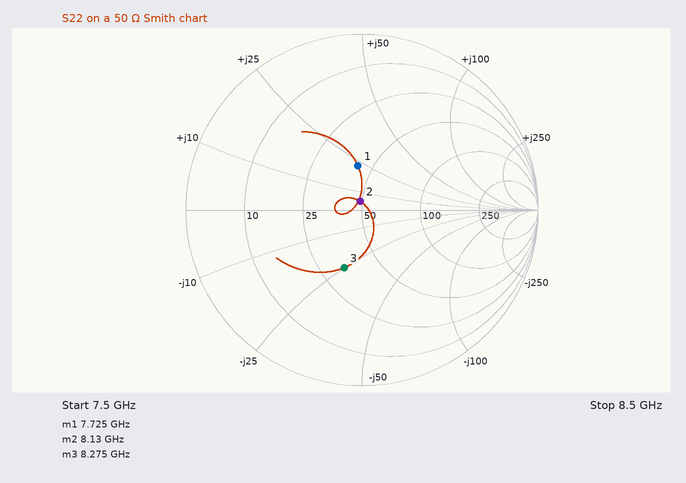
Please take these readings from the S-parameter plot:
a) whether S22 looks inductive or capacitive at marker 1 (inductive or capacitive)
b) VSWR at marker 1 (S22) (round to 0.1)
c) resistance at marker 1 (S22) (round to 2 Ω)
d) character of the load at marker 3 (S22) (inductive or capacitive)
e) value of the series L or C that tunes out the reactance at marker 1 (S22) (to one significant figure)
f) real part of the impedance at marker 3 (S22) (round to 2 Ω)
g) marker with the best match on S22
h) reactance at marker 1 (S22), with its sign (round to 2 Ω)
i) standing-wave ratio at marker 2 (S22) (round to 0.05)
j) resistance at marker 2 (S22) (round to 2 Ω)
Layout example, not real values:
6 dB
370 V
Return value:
inductive
1.7
42 Ω
capacitive
900 fF
34 Ω
marker 2
+22 Ω
1.10
48 Ω
